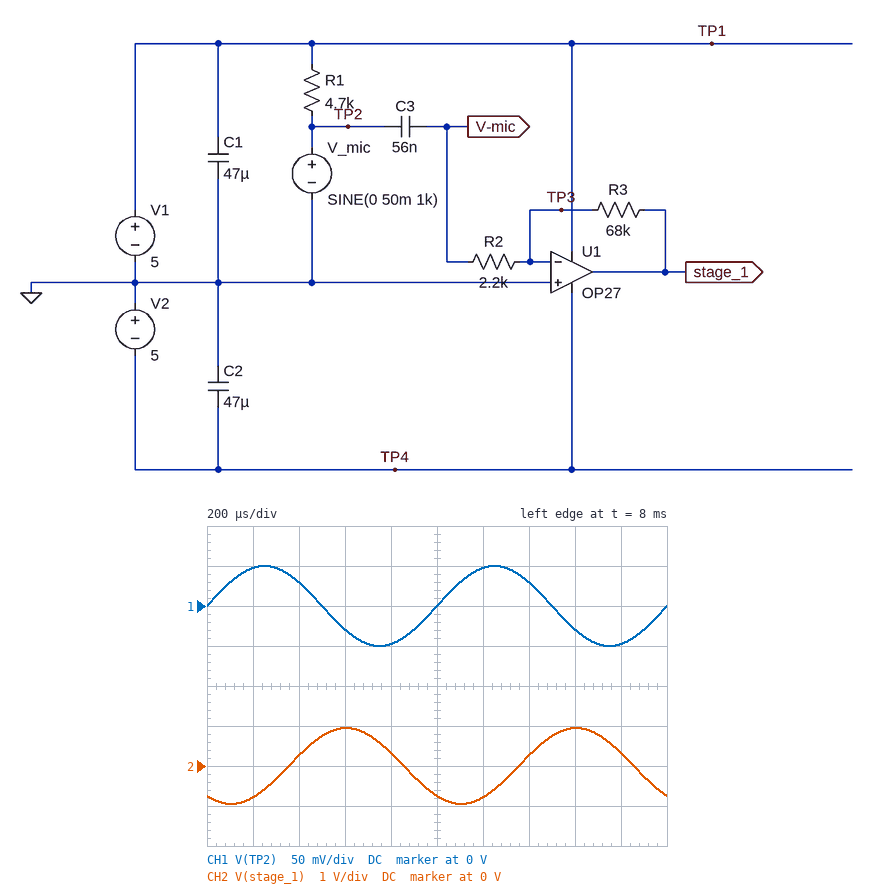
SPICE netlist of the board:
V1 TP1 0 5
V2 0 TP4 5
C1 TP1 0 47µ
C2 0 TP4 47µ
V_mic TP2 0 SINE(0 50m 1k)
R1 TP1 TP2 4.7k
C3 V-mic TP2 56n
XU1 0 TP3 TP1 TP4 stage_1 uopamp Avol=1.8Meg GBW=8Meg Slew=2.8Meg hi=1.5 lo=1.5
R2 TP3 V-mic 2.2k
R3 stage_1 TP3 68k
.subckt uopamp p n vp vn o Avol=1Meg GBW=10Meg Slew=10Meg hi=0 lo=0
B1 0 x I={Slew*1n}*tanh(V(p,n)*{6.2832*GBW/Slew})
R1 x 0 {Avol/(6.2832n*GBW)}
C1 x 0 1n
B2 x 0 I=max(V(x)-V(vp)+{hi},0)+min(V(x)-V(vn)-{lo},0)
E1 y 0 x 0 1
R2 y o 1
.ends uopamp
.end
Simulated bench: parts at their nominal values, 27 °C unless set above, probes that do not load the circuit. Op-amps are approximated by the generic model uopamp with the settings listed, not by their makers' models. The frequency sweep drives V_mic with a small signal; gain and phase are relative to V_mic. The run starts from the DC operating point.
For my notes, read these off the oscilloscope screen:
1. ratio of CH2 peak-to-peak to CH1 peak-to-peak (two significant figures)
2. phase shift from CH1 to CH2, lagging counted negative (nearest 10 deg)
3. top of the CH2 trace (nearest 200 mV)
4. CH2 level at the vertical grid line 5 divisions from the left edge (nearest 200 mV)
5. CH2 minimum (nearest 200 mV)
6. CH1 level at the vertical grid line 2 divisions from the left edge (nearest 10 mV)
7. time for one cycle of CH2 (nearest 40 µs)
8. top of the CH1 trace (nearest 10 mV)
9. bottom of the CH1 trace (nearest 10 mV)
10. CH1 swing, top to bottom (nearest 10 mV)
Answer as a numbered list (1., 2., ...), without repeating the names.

1. 19
2. -130 deg
3. 1.0 V
4. -800 mV
5. -1.0 V
6. 30 mV
7. 1.00 ms
8. 50 mV
9. -50 mV
10. 100 mV
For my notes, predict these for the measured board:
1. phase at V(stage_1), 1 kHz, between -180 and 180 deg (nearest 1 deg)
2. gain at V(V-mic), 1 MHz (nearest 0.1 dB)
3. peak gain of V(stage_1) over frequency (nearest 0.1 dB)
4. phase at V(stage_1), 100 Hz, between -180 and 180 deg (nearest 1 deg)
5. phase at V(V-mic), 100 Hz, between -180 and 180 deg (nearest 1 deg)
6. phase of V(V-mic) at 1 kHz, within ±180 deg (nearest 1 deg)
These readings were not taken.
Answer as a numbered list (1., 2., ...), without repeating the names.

1. -128 deg
2. 0 dB
3. 29.8 dB
4. -94 deg
5. 86 deg
6. 52 deg
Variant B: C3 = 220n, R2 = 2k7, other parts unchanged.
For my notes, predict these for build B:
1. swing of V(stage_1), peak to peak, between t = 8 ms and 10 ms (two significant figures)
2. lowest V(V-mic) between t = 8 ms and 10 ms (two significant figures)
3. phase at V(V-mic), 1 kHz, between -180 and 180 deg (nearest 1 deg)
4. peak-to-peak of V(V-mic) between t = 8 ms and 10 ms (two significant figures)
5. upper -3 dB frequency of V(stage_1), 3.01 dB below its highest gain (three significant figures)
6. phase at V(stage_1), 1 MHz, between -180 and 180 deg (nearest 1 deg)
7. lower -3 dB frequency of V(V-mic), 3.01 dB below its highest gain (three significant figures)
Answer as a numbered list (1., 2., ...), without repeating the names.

1. 2.4 V
2. -48 mV
3. 15 deg
4. 97 mV
5. 306 kHz
6. 107 deg
7. 268 Hz
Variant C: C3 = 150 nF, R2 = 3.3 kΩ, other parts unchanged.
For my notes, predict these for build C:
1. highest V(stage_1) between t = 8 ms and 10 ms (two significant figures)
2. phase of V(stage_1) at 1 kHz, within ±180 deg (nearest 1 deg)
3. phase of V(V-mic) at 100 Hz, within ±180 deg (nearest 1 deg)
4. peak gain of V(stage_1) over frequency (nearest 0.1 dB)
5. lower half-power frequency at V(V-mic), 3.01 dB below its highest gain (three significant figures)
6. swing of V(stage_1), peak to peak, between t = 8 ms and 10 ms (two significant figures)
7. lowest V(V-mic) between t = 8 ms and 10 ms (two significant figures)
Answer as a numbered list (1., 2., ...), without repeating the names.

1. 980 mV
2. -162 deg
3. 73 deg
4. 26.3 dB
5. 322 Hz
6. 2.0 V
7. -48 mV
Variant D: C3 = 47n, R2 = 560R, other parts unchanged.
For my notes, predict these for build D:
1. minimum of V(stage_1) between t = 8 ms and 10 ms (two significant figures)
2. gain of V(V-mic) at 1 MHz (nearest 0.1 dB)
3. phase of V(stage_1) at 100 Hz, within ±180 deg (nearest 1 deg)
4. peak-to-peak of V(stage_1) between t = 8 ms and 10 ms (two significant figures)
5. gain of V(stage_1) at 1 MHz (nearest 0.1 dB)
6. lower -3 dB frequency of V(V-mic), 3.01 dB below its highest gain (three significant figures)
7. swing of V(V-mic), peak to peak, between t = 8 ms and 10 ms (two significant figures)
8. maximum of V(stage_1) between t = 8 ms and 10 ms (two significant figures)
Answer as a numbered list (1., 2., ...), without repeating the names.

1. -990 mV
2. 0 dB
3. -91 deg
4. 2.0 V
5. 18.0 dB
6. 6.20 kHz
7. 16 mV
8. 990 mV
